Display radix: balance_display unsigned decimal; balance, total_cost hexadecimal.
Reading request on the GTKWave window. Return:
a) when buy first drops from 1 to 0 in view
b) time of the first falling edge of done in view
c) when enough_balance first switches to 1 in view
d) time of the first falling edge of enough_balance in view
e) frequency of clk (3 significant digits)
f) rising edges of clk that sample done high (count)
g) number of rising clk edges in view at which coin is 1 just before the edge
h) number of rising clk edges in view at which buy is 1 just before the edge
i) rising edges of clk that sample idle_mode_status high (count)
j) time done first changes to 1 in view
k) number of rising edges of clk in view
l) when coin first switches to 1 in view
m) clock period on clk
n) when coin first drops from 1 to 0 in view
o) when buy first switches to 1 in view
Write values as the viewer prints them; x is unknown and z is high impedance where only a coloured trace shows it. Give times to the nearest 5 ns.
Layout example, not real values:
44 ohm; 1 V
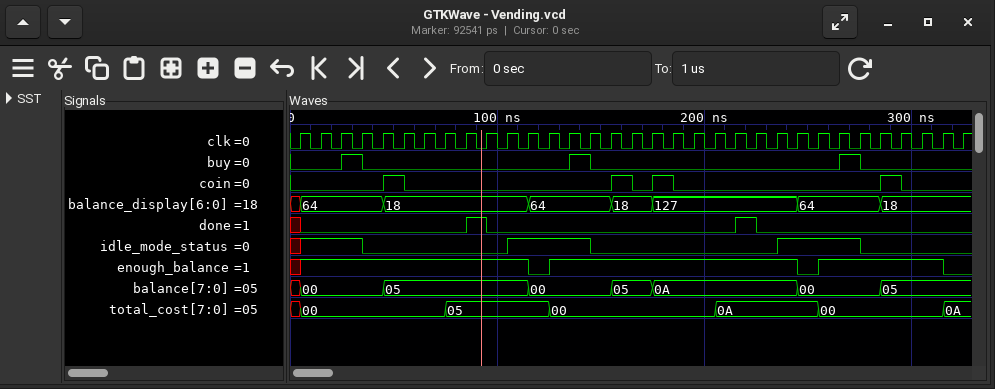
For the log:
35 ns; 95 ns; 5 ns; 115 ns; 100 MHz; 2; 4; 3; 11; 85 ns; 33; 45 ns; 10 ns; 55 ns; 25 ns
